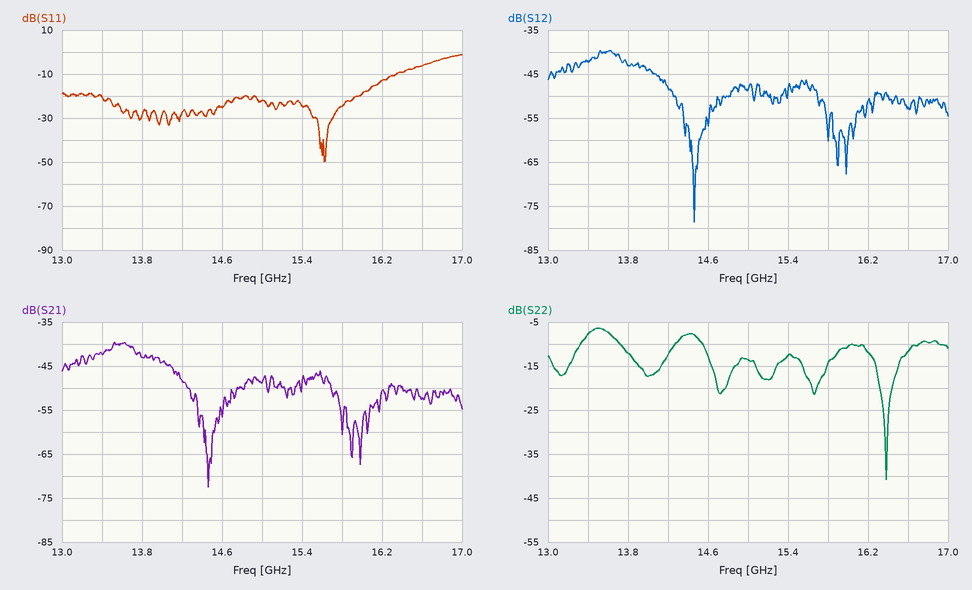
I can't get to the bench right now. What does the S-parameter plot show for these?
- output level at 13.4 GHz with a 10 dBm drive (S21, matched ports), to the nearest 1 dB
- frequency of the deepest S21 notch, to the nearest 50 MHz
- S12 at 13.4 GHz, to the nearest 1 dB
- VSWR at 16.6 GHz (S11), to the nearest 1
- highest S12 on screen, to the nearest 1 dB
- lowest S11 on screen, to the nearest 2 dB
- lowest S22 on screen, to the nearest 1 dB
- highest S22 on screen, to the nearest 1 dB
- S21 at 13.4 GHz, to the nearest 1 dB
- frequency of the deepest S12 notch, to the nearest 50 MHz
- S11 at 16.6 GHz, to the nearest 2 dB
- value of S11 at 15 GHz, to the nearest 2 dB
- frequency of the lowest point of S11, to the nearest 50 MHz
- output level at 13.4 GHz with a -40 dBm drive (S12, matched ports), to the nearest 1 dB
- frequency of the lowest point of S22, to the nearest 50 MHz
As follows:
-32 dBm
14.45 GHz
-42 dB
3
-40 dB
-50 dB
-41 dB
-6 dB
-42 dB
14.45 GHz
-6 dB
-22 dB
15.60 GHz
-82 dBm
16.40 GHz
